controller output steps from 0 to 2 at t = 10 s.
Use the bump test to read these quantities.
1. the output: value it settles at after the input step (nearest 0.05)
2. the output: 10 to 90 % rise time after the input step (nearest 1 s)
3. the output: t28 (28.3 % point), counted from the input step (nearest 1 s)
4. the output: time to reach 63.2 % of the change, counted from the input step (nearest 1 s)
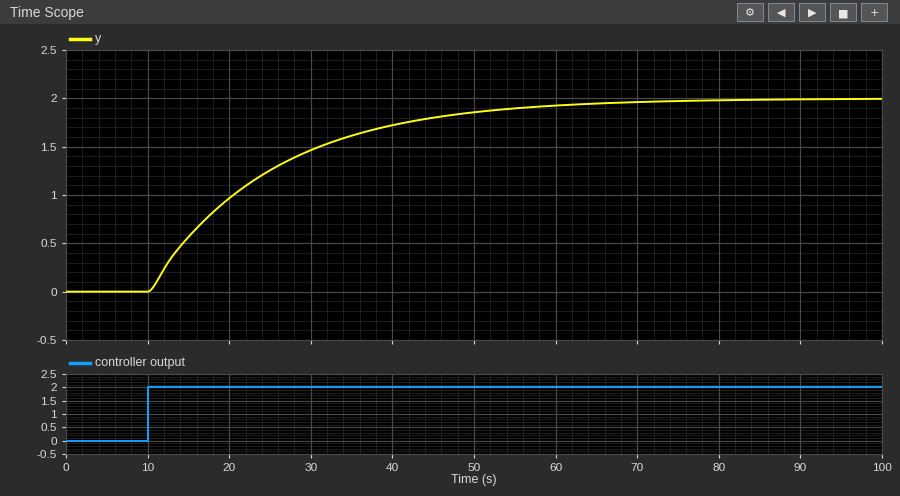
2.00
33 s
5 s
15 s
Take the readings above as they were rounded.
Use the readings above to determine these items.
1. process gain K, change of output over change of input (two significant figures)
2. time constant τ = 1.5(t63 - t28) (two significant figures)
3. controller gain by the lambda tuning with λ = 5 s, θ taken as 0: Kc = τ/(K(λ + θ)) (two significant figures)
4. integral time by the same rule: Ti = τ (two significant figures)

1.0
15 s
3.0
15 s
